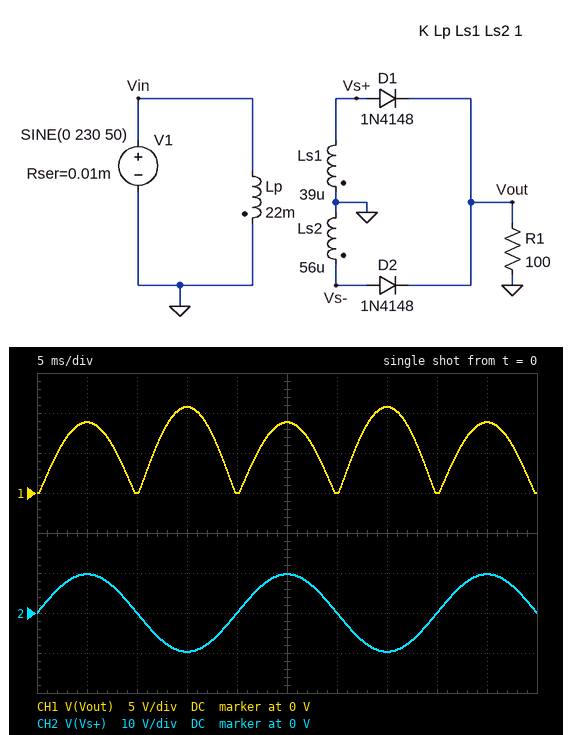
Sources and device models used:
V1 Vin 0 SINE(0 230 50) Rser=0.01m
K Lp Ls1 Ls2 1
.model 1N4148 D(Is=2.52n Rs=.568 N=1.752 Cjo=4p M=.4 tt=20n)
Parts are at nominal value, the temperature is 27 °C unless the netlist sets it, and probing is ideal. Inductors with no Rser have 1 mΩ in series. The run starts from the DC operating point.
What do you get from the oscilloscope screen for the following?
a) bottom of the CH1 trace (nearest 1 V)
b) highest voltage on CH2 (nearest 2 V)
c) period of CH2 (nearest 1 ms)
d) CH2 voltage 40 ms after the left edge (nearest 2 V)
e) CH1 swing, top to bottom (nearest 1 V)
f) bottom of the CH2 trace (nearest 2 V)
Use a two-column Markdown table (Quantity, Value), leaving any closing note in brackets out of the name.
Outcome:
| Quantity | Value |
|---|---|
| bottom of the CH1 trace | 0 V |
| highest voltage on CH2 | 10 V |
| period of CH2 | 20 ms |
| CH2 voltage 40 ms after the left edge | 0 V |
| CH1 swing, top to bottom | 11 V |
| bottom of the CH2 trace | -10 V |
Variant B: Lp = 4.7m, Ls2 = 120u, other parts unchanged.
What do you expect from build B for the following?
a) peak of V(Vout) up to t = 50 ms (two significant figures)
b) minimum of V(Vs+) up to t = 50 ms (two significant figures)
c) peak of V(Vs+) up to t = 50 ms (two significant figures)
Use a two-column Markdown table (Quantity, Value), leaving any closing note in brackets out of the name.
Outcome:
| Quantity | Value |
|---|---|
| peak of V(Vout) up to t = 50 ms | 36 V |
| minimum of V(Vs+) up to t = 50 ms | -21 V |
| peak of V(Vs+) up to t = 50 ms | 21 V |
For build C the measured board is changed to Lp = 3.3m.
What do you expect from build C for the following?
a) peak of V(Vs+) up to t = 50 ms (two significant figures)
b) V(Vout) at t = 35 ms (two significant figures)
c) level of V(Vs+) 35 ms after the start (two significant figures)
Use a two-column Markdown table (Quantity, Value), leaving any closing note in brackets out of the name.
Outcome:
| Quantity | Value |
|---|---|
| peak of V(Vs+) up to t = 50 ms | 25 V |
| V(Vout) at t = 35 ms | 29 V |
| level of V(Vs+) 35 ms after the start | -25 V |
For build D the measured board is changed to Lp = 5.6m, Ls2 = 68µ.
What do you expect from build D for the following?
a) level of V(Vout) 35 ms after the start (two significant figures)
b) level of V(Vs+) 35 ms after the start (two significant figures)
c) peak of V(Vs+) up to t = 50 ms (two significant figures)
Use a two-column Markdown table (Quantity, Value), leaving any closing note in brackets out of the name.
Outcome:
| Quantity | Value |
|---|---|
| level of V(Vout) 35 ms after the start | 24 V |
| level of V(Vs+) 35 ms after the start | -19 V |
| peak of V(Vs+) up to t = 50 ms | 19 V |
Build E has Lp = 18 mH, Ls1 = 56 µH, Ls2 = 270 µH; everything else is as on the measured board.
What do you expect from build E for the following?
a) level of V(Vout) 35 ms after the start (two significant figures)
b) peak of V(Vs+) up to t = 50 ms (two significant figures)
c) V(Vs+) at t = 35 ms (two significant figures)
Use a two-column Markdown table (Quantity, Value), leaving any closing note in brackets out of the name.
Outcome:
| Quantity | Value |
|---|---|
| level of V(Vout) 35 ms after the start | 27 V |
| peak of V(Vs+) up to t = 50 ms | 13 V |
| V(Vs+) at t = 35 ms | -13 V |
